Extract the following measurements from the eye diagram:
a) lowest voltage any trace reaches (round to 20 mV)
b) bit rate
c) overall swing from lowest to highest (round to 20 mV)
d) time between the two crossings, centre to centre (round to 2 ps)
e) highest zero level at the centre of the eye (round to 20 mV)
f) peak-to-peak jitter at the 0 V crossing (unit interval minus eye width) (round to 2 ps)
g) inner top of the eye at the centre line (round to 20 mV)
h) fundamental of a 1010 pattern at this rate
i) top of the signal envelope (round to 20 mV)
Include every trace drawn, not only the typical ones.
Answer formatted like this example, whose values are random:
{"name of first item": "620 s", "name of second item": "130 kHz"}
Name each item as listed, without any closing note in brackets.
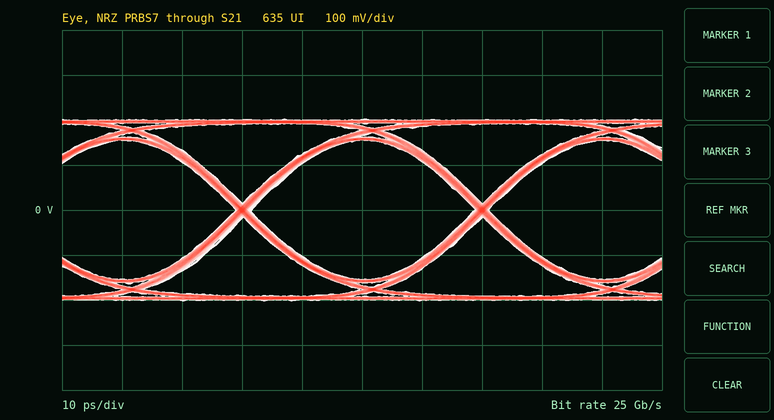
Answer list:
{"lowest voltage any trace reaches": "-200 mV", "bit rate": "25 Gb/s", "overall swing from lowest to highest": "400 mV", "time between the two crossings, centre to centre": "40 ps", "highest zero level at the centre of the eye": "-160 mV", "peak-to-peak jitter at the 0 V crossing (unit interval minus eye width)": "2 ps", "inner top of the eye at the centre line": "160 mV", "fundamental of a 1010 pattern at this rate": "12.5 GHz", "top of the signal envelope": "200 mV"}
